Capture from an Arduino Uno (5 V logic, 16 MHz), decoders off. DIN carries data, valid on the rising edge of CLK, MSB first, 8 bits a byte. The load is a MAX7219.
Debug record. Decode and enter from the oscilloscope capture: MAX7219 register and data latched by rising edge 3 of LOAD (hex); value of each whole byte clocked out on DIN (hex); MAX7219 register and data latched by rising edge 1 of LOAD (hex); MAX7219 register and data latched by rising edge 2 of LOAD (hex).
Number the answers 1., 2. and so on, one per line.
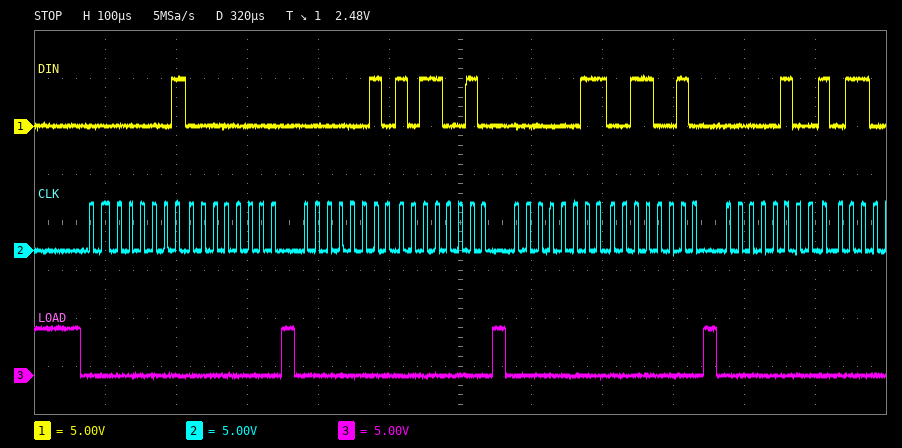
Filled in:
1. register 0x3, data 0x32
2. 0x01 0x00 0x02 0xB2 0x03 0x32 0x04
3. register 0x1, data 0x00
4. register 0x2, data 0xB2
